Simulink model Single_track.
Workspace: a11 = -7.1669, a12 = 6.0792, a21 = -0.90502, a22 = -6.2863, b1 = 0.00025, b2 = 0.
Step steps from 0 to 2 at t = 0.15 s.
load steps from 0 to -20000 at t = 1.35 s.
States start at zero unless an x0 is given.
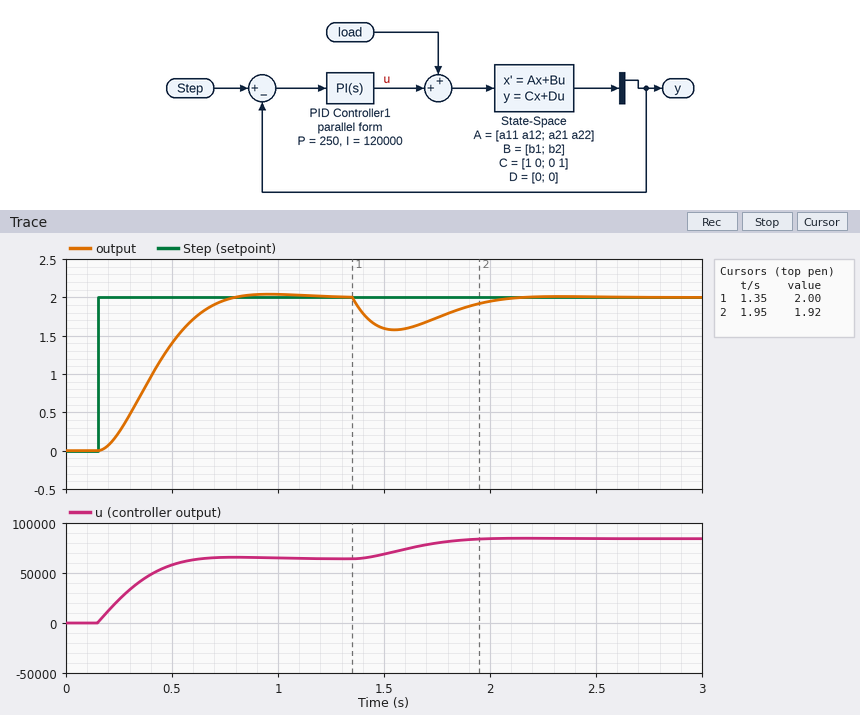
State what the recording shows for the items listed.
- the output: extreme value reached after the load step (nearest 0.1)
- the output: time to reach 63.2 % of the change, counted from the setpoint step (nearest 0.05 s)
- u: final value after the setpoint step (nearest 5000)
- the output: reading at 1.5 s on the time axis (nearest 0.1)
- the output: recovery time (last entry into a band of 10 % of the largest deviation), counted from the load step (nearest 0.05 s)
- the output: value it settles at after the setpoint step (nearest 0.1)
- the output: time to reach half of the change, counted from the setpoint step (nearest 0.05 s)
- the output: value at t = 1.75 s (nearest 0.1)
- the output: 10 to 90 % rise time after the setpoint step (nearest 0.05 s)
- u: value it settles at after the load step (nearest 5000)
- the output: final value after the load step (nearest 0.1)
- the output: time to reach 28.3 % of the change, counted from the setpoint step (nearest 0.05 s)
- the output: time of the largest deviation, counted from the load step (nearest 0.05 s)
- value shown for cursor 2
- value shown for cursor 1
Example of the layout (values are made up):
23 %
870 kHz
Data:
1.6
0.30 s
65000
1.6
0.65 s
2.0
0.25 s
1.7
0.40 s
85000
2.0
0.15 s
0.20 s
1.92
2.00
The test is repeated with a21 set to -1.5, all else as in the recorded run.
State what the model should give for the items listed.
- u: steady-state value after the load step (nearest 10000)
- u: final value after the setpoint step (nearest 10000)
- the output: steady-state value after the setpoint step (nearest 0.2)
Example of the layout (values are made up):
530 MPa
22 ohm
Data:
90000
70000
2.0
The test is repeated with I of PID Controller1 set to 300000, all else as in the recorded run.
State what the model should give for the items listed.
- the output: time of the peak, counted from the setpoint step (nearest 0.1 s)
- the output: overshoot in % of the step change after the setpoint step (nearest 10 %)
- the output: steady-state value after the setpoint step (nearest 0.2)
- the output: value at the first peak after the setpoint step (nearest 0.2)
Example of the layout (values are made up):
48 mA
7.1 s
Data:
0.4 s
20 %
2.0
2.4
